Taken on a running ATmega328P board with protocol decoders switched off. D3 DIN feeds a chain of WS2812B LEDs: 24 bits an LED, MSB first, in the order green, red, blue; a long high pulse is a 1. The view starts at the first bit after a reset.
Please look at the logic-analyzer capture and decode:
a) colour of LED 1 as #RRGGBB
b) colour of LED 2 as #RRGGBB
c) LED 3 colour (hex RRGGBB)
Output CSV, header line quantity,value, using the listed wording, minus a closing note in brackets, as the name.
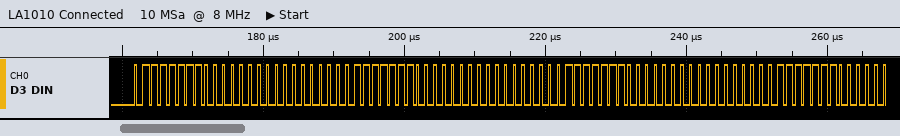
quantity,value
colour of LED 1 as #RRGGBB,#007F00
colour of LED 2 as #RRGGBB,#007F00
LED 3 colour,#007F00
